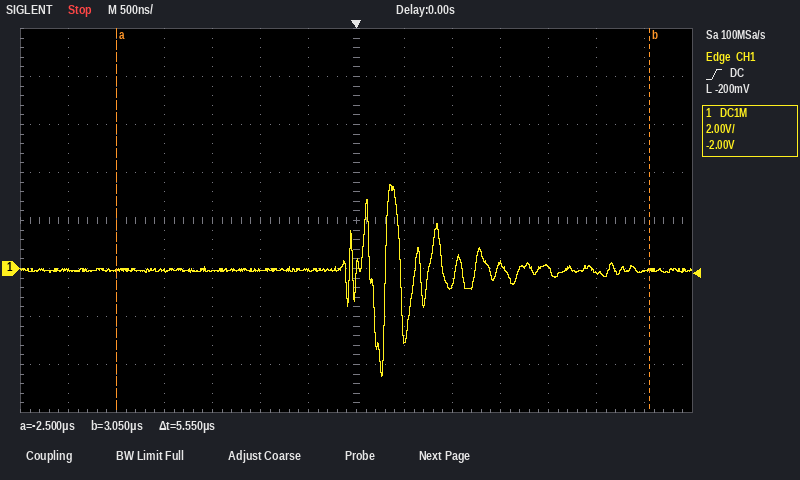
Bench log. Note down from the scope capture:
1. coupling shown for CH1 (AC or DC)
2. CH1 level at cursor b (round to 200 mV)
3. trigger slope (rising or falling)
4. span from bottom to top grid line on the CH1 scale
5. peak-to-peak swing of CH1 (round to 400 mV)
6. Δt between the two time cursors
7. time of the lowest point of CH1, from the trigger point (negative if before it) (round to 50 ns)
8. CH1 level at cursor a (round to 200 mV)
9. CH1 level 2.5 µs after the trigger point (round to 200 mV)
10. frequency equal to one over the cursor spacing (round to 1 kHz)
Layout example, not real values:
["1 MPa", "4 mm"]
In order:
["DC", "0.0 V", "rising", "16 V", "8.0 V", "5.55 µs", "+250 ns", "0.0 V", "-200 mV", "180 kHz"]
